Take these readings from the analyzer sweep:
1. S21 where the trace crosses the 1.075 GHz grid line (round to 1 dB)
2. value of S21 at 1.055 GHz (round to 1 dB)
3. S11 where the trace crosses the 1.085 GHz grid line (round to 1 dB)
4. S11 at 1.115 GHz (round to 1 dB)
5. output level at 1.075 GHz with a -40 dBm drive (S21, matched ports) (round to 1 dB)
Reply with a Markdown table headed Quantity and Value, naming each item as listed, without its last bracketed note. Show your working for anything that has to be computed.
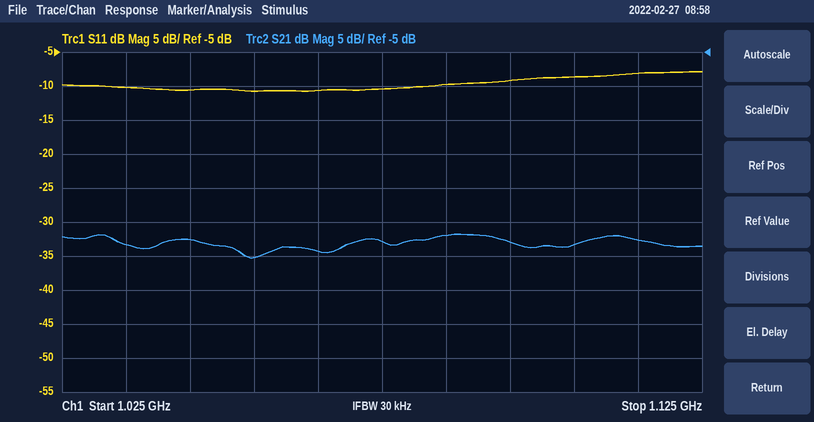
| Quantity | Value |
|---|---|
| S21 where the trace crosses the 1.075 GHz grid line | -33 dB |
| value of S21 at 1.055 GHz | -35 dB |
| S11 where the trace crosses the 1.085 GHz grid line | -10 dB |
| S11 at 1.115 GHz | -8 dB |
| output level at 1.075 GHz with a -40 dBm drive (S21, matched ports) | -40 dBm + (-33 dB) = -73 dBm |
